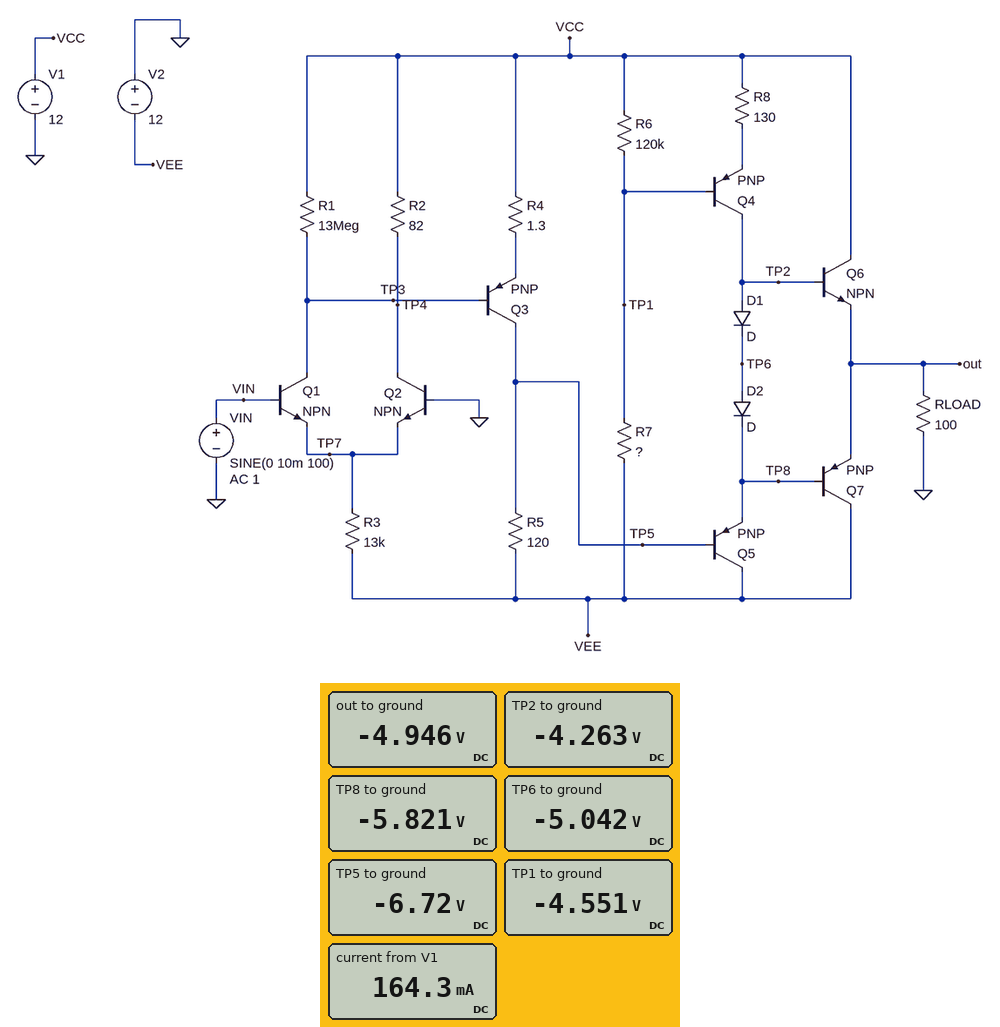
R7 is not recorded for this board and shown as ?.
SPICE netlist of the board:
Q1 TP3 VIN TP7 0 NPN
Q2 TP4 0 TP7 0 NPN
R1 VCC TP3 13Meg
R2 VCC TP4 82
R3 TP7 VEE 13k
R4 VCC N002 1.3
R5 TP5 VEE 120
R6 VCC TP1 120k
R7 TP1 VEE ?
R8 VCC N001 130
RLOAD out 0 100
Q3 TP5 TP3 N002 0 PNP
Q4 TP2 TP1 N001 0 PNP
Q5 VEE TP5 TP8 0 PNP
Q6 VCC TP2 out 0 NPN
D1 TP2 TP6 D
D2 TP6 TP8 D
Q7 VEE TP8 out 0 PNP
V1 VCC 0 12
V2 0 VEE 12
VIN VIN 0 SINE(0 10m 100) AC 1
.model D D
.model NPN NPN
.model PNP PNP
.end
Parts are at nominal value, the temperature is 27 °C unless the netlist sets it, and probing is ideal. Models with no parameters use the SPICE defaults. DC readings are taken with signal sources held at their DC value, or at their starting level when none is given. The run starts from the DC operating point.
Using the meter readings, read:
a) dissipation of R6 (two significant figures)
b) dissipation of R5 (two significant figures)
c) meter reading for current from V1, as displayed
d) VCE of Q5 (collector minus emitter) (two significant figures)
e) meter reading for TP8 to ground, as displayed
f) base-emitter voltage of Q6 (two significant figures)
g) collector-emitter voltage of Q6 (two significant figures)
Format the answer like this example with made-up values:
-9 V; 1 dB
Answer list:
2.3 mW; 230 mW; 164.3 mA; -6.2 V; -5.821 V; 680 mV; 17 V
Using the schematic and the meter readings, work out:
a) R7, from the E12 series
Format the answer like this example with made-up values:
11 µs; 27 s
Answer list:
5.6 kΩ
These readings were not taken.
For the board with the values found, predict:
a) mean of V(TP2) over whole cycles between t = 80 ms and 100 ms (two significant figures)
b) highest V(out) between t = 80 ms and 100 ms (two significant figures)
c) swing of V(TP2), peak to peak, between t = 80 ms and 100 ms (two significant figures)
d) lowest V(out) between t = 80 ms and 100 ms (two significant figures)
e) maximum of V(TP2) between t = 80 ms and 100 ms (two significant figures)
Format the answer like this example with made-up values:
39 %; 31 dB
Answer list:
-4.3 V; -4.0 V; 2.0 V; -5.9 V; -3.3 V
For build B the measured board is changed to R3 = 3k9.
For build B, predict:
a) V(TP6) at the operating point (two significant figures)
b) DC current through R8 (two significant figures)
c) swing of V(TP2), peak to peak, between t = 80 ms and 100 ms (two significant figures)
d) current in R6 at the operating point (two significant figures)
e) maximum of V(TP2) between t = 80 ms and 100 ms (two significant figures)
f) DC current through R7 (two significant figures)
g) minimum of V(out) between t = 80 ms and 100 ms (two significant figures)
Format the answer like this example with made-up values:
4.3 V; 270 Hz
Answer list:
6.7 V; 34 mA; 6.3 V; 44 µA; 11 V; 3.3 mA; 3.4 V
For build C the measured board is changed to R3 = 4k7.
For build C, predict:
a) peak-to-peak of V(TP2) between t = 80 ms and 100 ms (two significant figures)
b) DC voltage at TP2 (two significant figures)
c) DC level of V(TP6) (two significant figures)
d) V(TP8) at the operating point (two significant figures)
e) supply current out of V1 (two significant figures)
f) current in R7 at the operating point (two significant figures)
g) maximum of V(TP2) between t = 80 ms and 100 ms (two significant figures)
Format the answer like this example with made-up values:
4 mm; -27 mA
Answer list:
5.3 V; 4.6 V; 3.9 V; 3.1 V; 210 mA; 2.8 mA; 7.3 V
